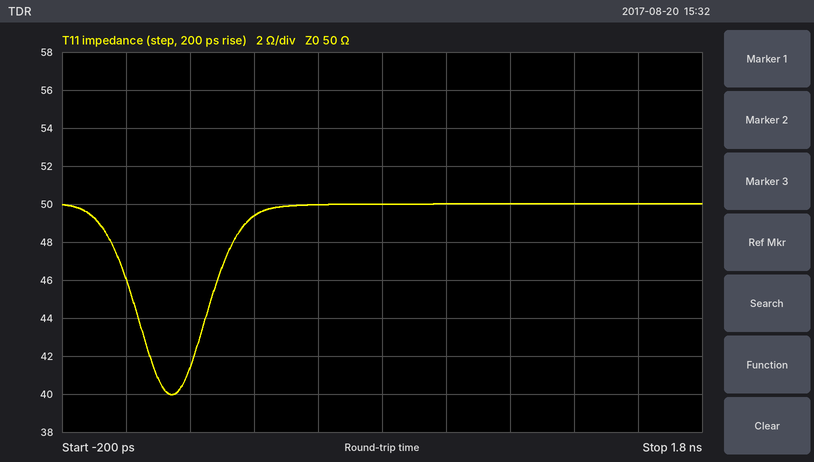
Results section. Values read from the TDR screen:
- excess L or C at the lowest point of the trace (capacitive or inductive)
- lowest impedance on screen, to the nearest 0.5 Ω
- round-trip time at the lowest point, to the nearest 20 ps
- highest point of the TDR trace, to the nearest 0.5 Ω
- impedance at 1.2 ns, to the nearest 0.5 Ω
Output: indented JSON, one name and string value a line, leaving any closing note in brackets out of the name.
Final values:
{
  "excess L or C at the lowest point of the trace": "capacitive",
  "lowest impedance on screen, to the nearest 0.5 Ω": "40.0 Ω",
  "round-trip time at the lowest point, to the nearest 20 ps": "140 ps",
  "highest point of the TDR trace, to the nearest 0.5 Ω": "50.0 Ω",
  "impedance at 1.2 ns, to the nearest 0.5 Ω": "50.0 Ω"
}
